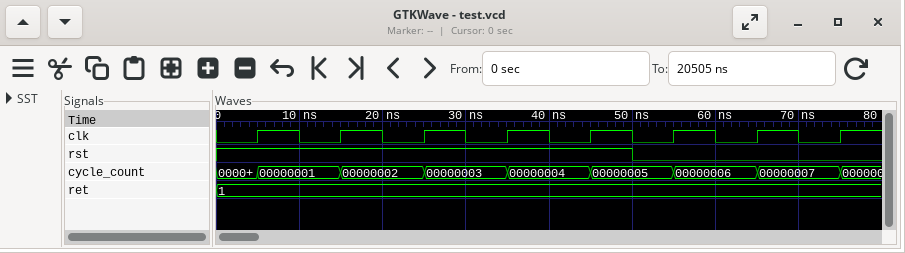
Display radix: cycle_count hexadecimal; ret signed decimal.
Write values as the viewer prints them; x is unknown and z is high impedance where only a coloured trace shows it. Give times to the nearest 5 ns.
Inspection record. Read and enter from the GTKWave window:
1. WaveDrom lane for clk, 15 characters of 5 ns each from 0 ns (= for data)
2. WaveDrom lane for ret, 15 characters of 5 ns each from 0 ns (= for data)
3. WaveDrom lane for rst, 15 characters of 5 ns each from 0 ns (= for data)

{name: 'clk', wave: '010101010101010'}
{name: 'ret', wave: '=..............', data: '1'}
{name: 'rst', wave: '1.........0....'}
